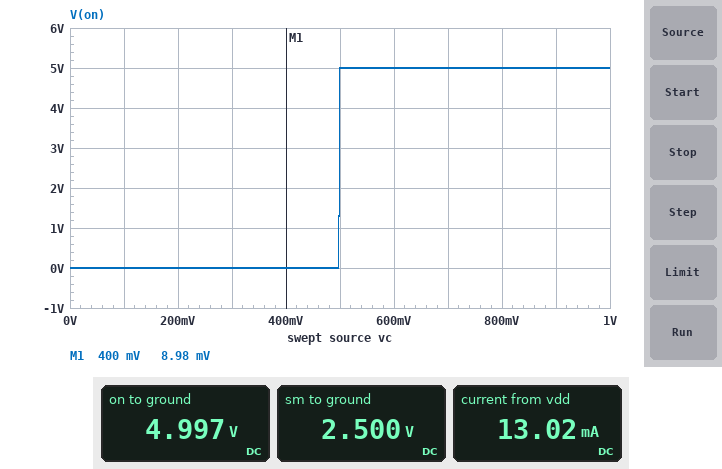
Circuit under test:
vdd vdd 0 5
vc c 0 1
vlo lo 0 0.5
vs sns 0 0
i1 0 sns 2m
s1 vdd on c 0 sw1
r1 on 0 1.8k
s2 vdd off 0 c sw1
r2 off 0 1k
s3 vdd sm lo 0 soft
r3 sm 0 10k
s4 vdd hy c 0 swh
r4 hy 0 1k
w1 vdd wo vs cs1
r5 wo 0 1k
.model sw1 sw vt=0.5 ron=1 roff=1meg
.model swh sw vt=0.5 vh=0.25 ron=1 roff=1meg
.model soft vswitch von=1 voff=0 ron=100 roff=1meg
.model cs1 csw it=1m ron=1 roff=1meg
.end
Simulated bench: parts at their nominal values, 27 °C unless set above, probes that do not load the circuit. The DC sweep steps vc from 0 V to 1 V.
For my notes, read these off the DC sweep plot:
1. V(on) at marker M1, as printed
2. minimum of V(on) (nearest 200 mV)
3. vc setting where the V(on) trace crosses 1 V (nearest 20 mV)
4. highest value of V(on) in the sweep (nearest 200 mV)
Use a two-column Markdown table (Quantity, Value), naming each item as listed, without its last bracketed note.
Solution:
| Quantity | Value |
|---|---|
| V(on) at marker M1, as printed | 8.98 mV |
| minimum of V(on) | 0 V |
| vc setting where the V(on) trace crosses 1 V | 500 mV |
| highest value of V(on) in the sweep | 5.0 V |
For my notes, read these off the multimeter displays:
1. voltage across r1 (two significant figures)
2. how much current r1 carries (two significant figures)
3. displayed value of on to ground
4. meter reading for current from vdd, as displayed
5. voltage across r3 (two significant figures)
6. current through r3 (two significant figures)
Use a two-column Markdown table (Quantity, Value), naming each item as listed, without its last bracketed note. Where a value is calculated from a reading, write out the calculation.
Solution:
| Quantity | Value |
|---|---|
| voltage across r1 | 4.997 V = 5.0 V |
| how much current r1 carries | (4.997 V) / 1.8 kΩ = 2.8 mA |
| displayed value of on to ground | 4.997 V |
| meter reading for current from vdd, as displayed | 13.02 mA |
| voltage across r3 | 2.5 V = 2.5 V |
| current through r3 | (2.5 V) / 10 kΩ = 250 µA |
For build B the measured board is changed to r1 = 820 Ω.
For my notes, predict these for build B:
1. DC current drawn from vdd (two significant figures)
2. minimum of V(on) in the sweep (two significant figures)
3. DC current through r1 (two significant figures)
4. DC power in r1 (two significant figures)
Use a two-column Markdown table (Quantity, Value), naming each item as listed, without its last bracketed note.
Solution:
| Quantity | Value |
|---|---|
| DC current drawn from vdd | 16 mA |
| minimum of V(on) in the sweep | 4.1 mV |
| DC current through r1 | 6.1 mA |
| DC power in r1 | 30 mW |
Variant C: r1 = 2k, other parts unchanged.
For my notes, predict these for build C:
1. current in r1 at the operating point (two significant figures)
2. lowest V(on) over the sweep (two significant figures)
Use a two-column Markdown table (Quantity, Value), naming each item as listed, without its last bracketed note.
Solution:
| Quantity | Value |
|---|---|
| current in r1 at the operating point | 2.5 mA |
| lowest V(on) over the sweep | 10 mV |
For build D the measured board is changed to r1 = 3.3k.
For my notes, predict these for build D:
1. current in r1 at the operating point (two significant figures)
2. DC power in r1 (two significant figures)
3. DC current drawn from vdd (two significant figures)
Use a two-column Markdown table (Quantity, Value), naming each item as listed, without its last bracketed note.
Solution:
| Quantity | Value |
|---|---|
| current in r1 at the operating point | 1.5 mA |
| DC power in r1 | 7.6 mW |
| DC current drawn from vdd | 12 mA |
